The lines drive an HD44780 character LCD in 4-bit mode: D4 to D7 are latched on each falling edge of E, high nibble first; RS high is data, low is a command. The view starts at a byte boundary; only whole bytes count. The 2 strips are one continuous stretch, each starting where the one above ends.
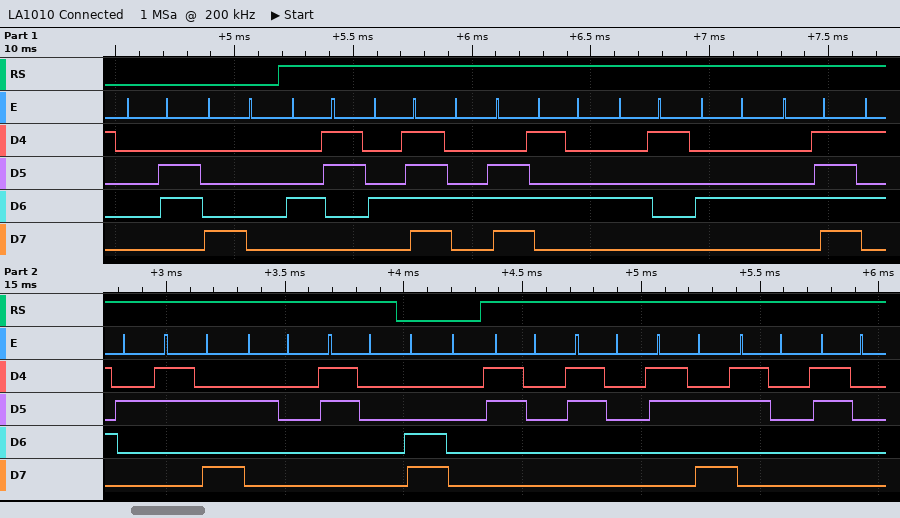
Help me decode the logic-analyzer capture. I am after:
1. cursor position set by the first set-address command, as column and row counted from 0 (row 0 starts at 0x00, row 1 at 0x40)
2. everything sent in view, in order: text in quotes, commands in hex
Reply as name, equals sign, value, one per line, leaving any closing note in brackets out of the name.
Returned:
cursor position set by the first set-address command, as column and row counted from 0 = column 0, row 0
everything sent in view, in order: text in quotes, commands in hex = 0x06 0x80 "CONTADOR: 0" 0xC0 "00:00"
